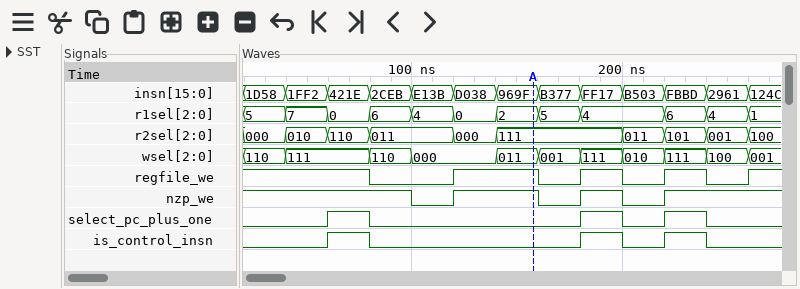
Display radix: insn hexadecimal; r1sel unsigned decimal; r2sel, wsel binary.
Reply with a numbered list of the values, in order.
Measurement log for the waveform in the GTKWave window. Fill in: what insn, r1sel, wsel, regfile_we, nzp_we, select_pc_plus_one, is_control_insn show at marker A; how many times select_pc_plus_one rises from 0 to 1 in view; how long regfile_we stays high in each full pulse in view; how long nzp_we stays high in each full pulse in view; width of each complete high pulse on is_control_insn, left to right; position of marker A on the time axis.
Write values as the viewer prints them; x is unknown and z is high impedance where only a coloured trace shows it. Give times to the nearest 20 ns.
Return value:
1. insn=969F, r1sel=2, wsel=011, regfile_we=1, nzp_we=1, select_pc_plus_one=0, is_control_insn=0
2. 3
3. 40 ns, 20 ns, 20 ns
4. 40 ns, 20 ns
5. 20 ns, 20 ns, 20 ns
6. 160 ns
